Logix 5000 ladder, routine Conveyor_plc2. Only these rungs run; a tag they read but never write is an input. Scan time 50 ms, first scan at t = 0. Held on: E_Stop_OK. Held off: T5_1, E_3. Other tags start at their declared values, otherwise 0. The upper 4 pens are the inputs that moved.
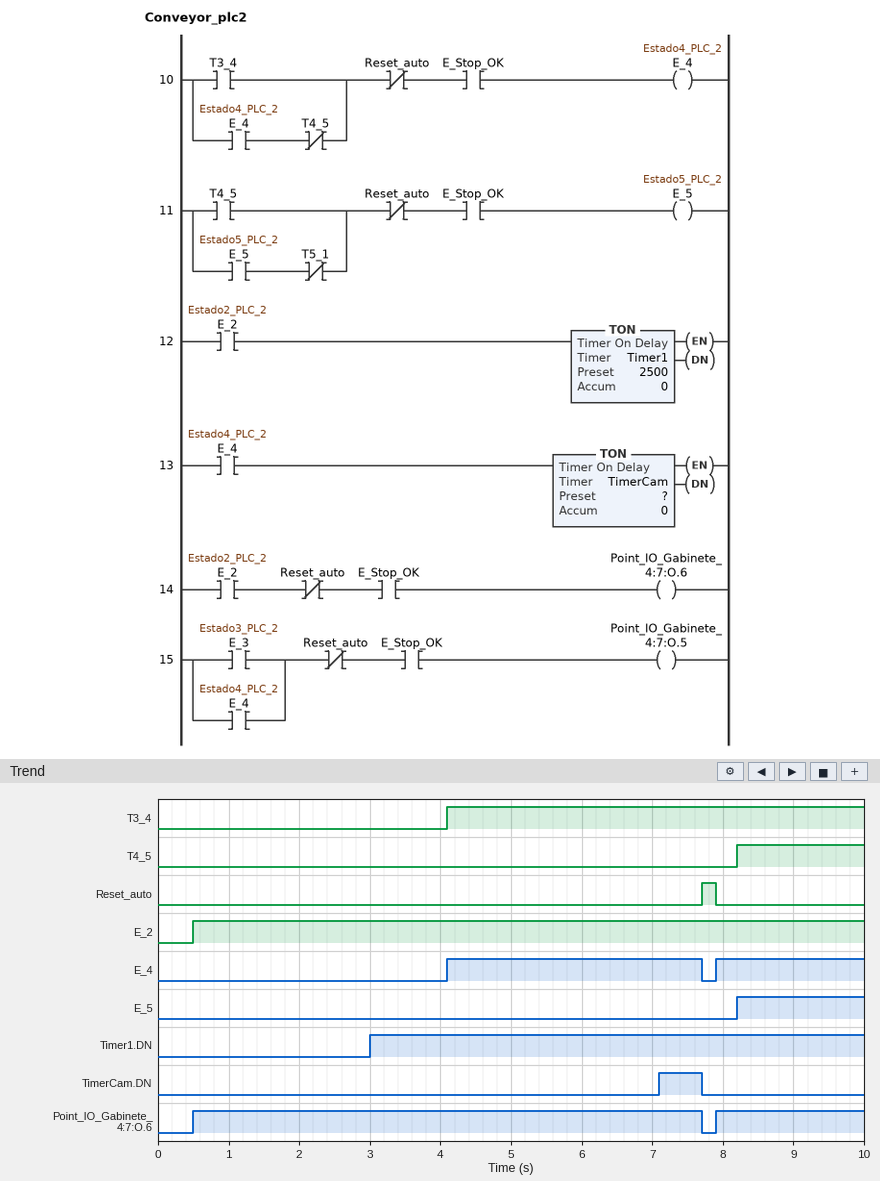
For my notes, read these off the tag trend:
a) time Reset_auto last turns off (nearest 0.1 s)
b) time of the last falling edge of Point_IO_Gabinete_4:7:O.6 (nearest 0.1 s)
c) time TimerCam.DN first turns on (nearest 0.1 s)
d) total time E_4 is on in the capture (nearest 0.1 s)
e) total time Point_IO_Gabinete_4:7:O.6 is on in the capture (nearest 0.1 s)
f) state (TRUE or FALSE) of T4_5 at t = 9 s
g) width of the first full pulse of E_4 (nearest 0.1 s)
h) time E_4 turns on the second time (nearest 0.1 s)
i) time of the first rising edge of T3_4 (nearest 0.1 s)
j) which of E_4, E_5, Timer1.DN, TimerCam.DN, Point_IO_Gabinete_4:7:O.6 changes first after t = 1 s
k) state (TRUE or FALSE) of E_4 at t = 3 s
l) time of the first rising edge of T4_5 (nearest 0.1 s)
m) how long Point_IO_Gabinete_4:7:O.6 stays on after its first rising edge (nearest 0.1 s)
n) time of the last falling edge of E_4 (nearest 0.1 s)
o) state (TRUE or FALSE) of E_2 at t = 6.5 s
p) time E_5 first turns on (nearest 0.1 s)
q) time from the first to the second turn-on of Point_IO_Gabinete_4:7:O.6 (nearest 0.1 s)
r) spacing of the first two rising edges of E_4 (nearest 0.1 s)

7.9 s
7.7 s
7.1 s
5.7 s
9.3 s
TRUE
3.6 s
7.9 s
4.1 s
Timer1.DN
FALSE
8.2 s
7.2 s
7.7 s
TRUE
8.2 s
7.4 s
3.8 s
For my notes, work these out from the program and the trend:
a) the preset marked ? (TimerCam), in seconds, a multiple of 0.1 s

3.0 s
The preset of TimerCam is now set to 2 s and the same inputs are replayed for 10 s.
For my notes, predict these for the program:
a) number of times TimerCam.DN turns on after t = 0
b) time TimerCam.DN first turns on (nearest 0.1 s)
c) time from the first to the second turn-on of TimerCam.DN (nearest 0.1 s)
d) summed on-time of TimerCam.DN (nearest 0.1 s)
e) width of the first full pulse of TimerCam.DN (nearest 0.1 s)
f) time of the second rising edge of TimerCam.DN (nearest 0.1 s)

2
6.1 s
3.8 s
1.7 s
1.6 s
9.9 s
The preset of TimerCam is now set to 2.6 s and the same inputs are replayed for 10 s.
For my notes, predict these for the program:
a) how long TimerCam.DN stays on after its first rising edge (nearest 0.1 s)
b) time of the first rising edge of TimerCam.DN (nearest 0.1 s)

1.0 s
6.7 s
